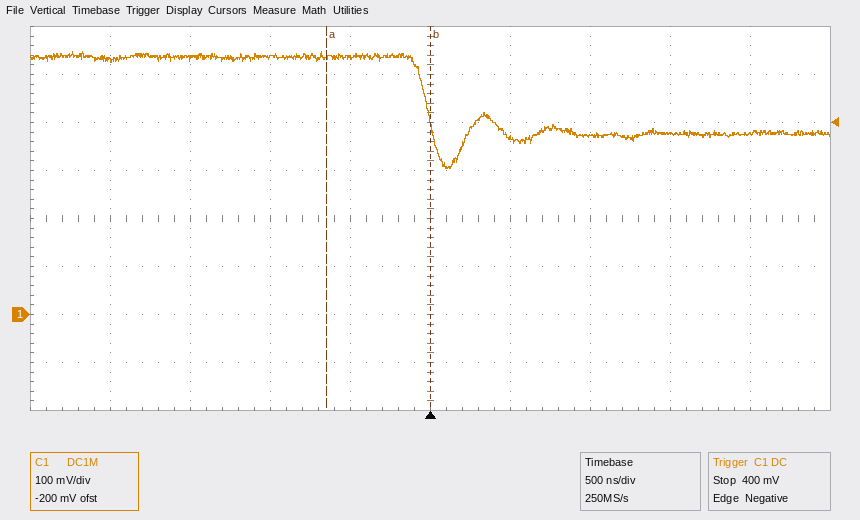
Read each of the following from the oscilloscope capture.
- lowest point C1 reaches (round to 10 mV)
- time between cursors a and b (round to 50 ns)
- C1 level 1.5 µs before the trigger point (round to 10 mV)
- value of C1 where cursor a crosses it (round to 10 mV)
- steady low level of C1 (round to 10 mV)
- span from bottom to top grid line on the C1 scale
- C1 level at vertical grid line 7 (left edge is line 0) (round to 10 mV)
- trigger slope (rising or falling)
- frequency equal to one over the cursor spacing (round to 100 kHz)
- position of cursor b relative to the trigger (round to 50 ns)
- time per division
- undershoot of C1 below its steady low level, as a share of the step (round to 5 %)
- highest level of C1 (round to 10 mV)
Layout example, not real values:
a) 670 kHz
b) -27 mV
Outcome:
a) 300 mV
b) 650 ns
c) 530 mV
d) 540 mV
e) 380 mV
f) 800 mV
g) 370 mV
h) falling
i) 1.5 MHz
j) 0 ns
k) 500 ns
l) 45 %
m) 550 mV
